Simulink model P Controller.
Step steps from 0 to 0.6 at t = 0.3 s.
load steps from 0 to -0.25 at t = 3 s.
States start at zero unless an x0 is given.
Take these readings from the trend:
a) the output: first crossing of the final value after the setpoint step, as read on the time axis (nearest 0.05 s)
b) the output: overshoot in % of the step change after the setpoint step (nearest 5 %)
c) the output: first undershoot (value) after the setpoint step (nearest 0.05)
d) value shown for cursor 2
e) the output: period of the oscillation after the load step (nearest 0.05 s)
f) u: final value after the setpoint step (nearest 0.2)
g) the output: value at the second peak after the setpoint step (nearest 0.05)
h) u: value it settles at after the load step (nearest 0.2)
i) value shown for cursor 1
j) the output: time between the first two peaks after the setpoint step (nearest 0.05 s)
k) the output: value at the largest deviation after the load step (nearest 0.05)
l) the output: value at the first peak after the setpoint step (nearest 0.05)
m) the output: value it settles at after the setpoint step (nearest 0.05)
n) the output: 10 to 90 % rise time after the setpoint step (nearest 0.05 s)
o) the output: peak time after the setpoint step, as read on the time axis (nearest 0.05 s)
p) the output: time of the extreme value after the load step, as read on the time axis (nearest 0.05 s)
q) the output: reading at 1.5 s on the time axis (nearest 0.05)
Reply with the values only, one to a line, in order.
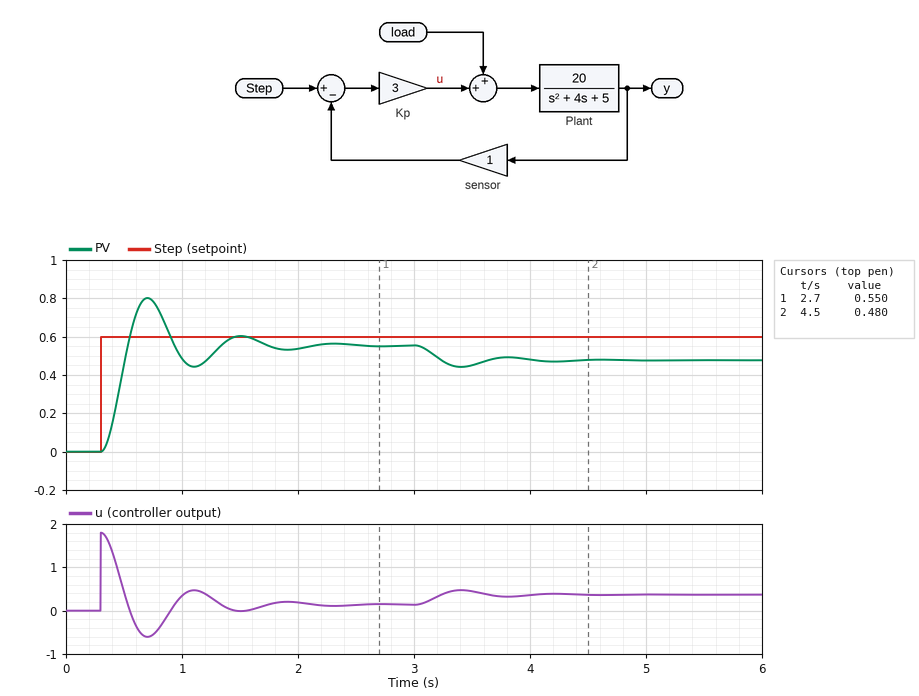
0.55 s
45 %
0.45
0.480
0.80 s
0.2
0.60
0.4
0.550
0.80 s
0.45
0.80
0.55
0.15 s
0.70 s
3.40 s
0.60
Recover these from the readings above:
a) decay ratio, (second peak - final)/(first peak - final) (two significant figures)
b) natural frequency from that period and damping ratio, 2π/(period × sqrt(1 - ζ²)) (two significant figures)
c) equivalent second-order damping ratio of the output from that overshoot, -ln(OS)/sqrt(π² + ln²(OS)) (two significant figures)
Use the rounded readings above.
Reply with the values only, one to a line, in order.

0.20
8.1 rad/s
0.25
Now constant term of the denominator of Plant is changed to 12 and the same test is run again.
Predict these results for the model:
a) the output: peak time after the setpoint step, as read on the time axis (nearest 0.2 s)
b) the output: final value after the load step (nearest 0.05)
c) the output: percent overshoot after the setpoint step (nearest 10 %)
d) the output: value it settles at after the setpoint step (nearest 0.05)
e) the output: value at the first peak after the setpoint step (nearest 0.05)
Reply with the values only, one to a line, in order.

0.6 s
0.45
50 %
0.50
0.75
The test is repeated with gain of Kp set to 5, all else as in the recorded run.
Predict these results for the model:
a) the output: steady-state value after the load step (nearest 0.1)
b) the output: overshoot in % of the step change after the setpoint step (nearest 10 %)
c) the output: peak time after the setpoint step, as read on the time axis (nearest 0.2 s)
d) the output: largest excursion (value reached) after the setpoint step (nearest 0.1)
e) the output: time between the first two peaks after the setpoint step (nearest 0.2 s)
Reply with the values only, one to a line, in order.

0.5
50 %
0.6 s
0.9
0.6 s
